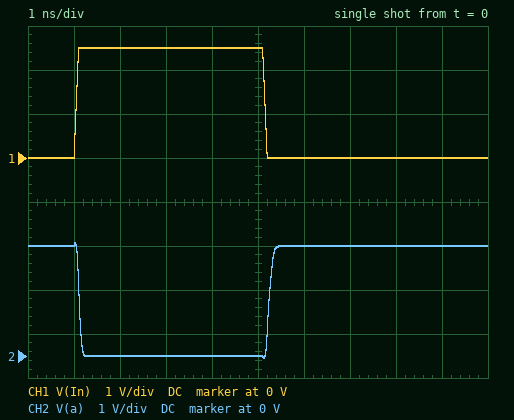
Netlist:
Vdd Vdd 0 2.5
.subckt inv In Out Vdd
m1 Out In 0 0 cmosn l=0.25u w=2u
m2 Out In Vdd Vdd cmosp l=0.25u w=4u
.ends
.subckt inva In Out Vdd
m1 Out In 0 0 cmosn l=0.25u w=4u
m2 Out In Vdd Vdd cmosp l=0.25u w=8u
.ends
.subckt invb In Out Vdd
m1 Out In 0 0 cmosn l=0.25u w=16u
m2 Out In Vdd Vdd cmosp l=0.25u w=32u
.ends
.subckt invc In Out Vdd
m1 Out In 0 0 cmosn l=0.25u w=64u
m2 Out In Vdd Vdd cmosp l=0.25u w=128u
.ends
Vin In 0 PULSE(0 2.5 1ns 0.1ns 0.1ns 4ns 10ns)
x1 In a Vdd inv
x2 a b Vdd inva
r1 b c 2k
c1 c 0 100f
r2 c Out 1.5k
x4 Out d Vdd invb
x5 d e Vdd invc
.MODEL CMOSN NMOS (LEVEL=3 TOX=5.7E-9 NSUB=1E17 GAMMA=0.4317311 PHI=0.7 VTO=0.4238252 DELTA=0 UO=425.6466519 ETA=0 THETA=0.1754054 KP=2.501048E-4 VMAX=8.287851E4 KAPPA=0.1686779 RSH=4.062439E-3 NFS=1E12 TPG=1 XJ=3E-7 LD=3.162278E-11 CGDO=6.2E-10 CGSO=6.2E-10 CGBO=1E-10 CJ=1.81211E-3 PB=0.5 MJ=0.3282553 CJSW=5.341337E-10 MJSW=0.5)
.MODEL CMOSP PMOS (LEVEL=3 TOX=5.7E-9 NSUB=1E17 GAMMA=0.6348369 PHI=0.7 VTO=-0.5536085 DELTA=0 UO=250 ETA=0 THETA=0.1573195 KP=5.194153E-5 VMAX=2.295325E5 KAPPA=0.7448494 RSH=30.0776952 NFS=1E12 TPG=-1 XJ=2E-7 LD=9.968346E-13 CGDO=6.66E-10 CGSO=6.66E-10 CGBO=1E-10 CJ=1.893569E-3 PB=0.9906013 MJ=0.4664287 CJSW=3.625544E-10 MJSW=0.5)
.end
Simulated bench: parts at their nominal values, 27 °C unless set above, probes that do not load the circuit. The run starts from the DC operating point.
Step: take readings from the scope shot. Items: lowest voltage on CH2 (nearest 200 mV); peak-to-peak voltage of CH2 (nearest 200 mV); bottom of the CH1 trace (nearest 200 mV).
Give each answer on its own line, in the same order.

0 V
2.6 V
0 V
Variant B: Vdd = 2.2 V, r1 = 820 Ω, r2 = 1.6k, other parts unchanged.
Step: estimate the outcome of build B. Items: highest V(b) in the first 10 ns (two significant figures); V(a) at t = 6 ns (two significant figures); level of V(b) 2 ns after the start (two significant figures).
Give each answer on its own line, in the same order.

2.3 V
2.2 V
2.1 V
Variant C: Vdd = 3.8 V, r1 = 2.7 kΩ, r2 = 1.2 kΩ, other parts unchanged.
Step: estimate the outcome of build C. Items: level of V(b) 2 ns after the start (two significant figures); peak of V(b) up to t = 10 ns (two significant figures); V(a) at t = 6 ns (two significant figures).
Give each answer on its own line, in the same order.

3.6 V
3.9 V
3.8 V
